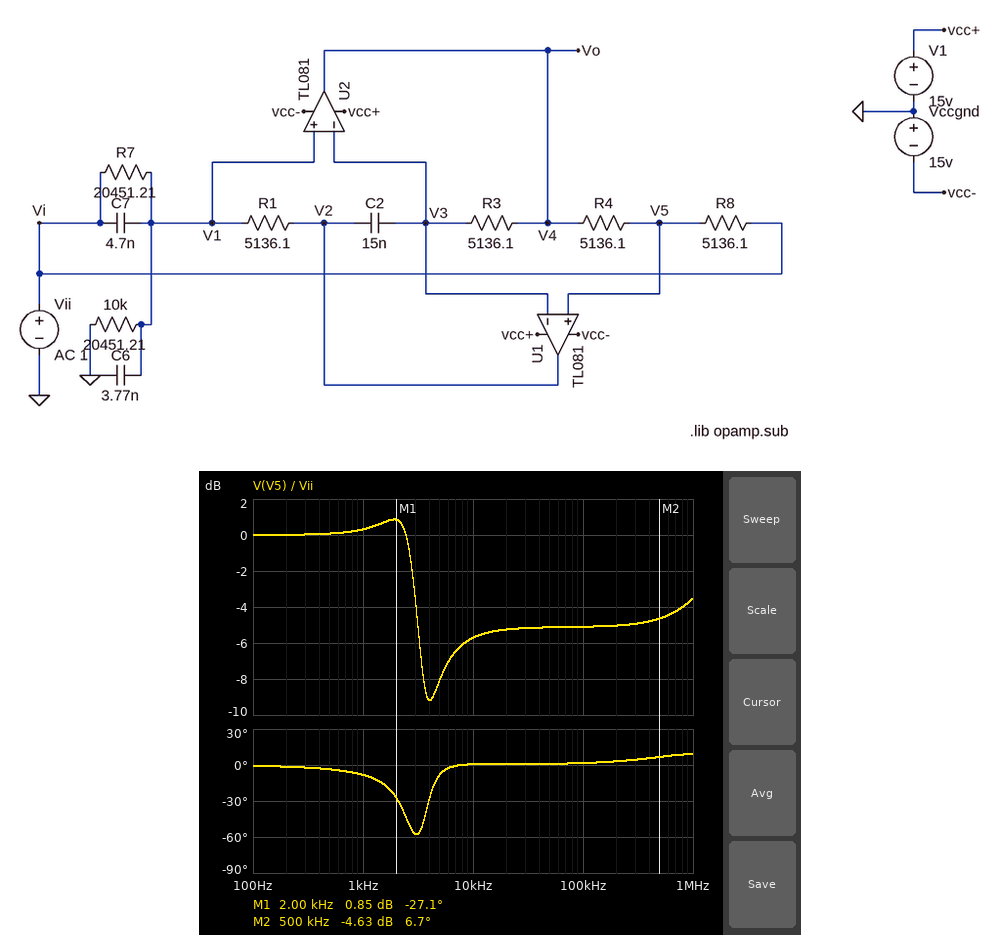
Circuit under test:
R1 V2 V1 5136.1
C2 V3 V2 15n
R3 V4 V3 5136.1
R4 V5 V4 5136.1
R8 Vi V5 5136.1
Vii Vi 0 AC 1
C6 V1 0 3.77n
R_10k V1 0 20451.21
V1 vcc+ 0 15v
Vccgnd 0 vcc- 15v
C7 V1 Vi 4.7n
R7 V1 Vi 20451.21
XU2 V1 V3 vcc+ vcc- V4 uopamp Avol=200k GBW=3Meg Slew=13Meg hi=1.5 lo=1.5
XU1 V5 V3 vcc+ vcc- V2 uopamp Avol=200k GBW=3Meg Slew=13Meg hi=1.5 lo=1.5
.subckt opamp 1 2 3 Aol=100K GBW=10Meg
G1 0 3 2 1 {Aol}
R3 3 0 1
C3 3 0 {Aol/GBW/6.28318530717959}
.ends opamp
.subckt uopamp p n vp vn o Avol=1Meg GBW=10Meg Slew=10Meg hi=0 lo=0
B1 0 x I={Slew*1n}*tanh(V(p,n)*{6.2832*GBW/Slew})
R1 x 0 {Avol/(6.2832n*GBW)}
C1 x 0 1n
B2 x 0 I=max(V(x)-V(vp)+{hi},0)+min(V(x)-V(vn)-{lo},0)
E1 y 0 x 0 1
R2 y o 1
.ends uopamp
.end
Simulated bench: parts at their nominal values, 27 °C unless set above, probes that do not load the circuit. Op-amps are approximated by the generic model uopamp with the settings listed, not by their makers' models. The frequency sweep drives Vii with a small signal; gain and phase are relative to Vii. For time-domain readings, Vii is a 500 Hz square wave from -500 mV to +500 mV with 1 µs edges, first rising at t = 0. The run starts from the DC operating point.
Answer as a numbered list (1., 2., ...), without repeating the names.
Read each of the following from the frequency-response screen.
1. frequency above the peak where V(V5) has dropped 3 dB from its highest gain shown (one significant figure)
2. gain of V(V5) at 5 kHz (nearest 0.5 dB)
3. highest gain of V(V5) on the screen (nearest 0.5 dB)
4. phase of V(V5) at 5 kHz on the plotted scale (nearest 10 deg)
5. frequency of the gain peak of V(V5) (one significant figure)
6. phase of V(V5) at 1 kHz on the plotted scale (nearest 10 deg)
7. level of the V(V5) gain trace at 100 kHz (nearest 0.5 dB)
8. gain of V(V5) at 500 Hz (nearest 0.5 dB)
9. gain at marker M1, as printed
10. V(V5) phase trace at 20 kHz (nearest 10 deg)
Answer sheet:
1. 3 kHz
2. -8.0 dB
3. 1.0 dB
4. -10 deg
5. 2 kHz
6. -10 deg
7. -5.0 dB
8. 0 dB
9. 0.85 dB
10. 0 deg
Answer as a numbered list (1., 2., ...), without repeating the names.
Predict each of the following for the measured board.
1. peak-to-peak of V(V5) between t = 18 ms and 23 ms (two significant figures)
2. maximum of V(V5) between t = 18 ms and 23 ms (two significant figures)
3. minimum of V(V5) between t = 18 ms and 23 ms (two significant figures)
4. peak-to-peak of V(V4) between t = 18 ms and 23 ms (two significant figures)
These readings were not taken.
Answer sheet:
1. 1.3 V
2. 650 mV
3. -650 mV
4. 1.6 V
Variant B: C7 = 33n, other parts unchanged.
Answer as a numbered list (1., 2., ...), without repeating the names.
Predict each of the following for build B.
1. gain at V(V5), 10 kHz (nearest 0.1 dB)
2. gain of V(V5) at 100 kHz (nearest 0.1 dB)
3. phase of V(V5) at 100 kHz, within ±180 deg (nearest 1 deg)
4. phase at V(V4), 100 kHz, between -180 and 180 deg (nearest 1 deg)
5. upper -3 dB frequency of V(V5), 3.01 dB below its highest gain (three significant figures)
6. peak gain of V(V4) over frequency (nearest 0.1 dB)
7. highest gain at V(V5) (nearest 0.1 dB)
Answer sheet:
1. -1.0 dB
2. -0.9 dB
3. 0 deg
4. 1 deg
5. 3.98 MHz
6. 0.9 dB
7. 0.2 dB
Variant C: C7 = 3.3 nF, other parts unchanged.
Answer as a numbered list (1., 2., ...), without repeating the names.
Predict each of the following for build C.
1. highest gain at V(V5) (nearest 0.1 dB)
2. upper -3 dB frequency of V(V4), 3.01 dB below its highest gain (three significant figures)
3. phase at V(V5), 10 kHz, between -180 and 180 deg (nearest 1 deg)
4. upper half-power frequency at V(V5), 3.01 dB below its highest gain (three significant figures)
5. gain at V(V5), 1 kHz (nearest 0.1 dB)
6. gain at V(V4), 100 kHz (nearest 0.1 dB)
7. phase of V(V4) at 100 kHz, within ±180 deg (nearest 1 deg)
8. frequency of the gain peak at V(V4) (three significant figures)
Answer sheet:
1. 1.0 dB
2. 3.64 kHz
3. -2 deg
4. 3.16 kHz
5. 0.3 dB
6. -22.8 dB
7. 152 deg
8. 2.62 kHz
